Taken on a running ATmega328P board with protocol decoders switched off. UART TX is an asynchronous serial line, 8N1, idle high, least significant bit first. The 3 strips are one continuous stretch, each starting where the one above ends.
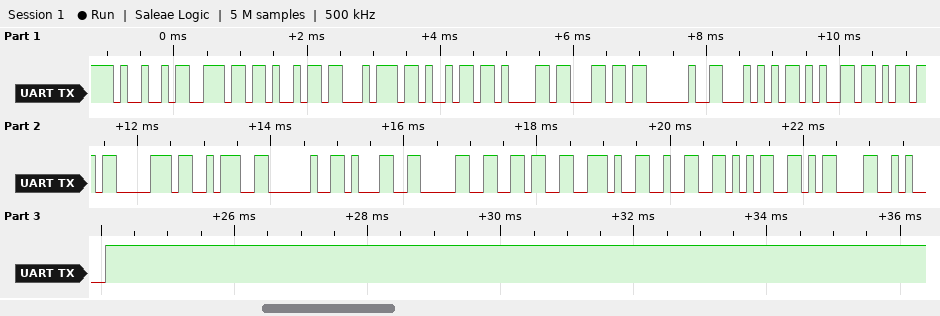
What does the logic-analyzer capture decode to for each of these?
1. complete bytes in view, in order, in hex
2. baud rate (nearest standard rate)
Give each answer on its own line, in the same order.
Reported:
49 6E 69 74 69 61 6C 20 54 65 6D 70 3A 20 31 30 36 2E 32 35 0D 0A
9600 baud
